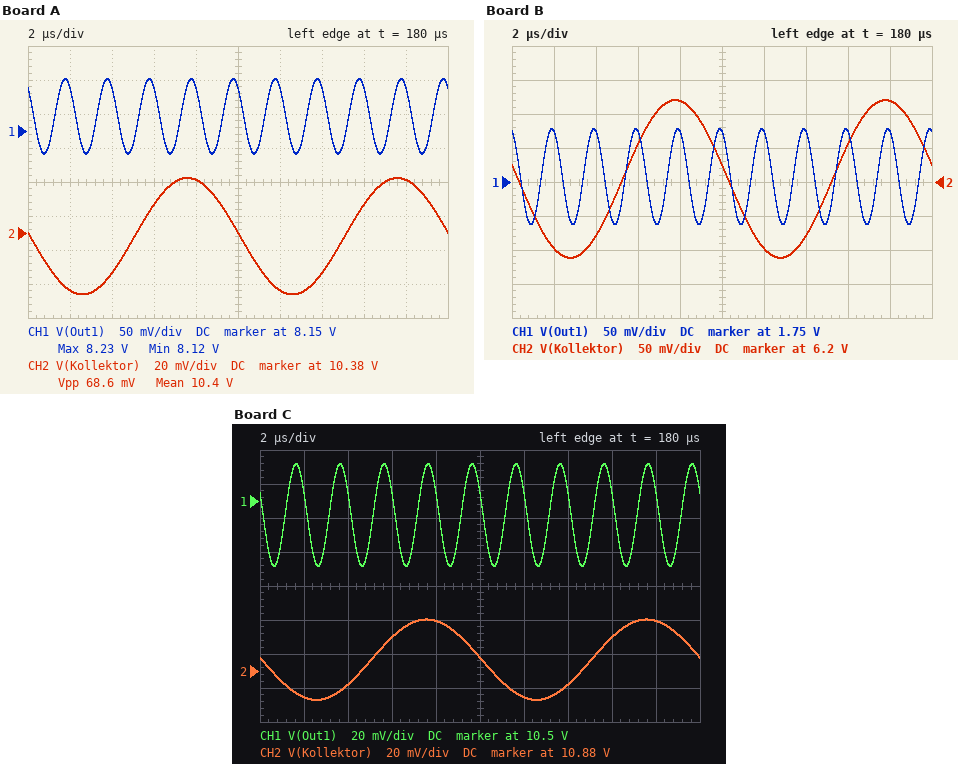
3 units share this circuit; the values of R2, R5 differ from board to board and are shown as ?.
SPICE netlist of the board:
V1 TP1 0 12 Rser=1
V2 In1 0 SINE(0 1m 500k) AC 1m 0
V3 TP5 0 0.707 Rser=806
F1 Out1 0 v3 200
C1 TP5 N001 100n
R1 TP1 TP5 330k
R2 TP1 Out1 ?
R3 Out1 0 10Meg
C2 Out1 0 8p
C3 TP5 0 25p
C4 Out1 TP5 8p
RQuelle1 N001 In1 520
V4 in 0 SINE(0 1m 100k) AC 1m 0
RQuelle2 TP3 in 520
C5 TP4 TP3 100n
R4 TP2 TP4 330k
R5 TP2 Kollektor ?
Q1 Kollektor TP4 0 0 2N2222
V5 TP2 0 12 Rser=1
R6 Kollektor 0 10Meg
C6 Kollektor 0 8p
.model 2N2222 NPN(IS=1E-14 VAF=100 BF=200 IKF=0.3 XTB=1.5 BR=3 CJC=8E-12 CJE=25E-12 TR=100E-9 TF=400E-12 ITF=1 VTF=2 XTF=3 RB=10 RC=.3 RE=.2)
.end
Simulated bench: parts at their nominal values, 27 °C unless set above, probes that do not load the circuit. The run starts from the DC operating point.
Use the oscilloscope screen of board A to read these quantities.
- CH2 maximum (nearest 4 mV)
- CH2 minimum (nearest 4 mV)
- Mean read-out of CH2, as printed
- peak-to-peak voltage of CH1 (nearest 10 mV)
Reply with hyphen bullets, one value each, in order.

- 10.412 V
- 10.344 V
- 10.4 V
- 110 mV
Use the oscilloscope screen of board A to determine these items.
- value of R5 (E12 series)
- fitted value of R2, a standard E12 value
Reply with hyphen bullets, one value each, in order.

- 220 Ω
- 560 Ω
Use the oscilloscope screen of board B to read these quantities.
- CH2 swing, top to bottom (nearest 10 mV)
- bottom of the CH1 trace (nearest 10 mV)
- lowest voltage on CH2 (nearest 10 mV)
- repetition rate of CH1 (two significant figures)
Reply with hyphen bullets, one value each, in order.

- 230 mV
- 1.69 V
- 6.09 V
- 500 kHz
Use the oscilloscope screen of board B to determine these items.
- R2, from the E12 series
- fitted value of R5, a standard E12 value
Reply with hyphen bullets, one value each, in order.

- 1.5 kΩ
- 820 Ω
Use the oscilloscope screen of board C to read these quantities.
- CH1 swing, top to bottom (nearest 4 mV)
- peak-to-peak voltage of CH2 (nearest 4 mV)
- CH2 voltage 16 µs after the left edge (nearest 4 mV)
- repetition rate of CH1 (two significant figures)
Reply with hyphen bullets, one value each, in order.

- 60 mV
- 48 mV
- 10.900 V
- 500 kHz
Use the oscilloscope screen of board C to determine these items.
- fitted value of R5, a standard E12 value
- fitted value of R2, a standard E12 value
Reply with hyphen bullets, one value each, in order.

- 150 Ω
- 220 Ω
